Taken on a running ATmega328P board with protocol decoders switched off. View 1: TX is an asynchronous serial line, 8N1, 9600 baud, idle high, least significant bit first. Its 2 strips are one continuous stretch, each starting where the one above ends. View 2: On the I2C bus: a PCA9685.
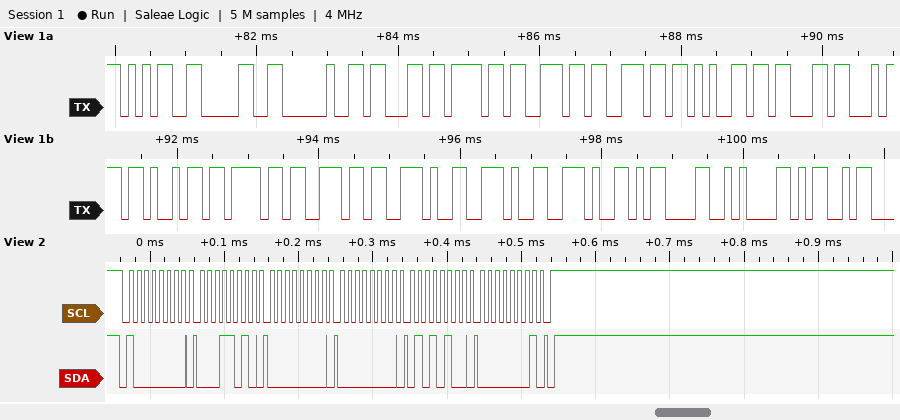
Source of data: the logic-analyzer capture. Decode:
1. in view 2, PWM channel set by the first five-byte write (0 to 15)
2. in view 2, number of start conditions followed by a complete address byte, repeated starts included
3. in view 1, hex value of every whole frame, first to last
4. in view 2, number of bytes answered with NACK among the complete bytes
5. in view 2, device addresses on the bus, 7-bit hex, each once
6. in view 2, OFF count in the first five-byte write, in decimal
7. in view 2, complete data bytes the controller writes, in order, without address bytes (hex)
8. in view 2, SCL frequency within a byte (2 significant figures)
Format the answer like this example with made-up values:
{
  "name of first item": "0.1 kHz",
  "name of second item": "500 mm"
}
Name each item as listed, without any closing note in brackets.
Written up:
{
  "in view 2, PWM channel set by the first five-byte write": "5",
  "in view 2, number of start conditions followed by a complete address byte, repeated starts included": "1",
  "in view 1, hex value of every whole frame, first to last": "0x35 0x30 0x20 0x63 0x6F 0x6E 0x6E 0x65 0x63 0x74 0x69 0x6F 0x6E 0x2E 0x2E 0x2E 0x0D 0x0A 0x4D",
  "in view 2, number of bytes answered with NACK among the complete bytes": "0",
  "in view 2, device addresses on the bus, 7-bit hex, each once": "0x40",
  "in view 2, OFF count in the first five-byte write, in decimal": "340",
  "in view 2, complete data bytes the controller writes, in order, without address bytes": "1A 00 00 54 01",
  "in view 2, SCL frequency within a byte": "100 kHz"
}
